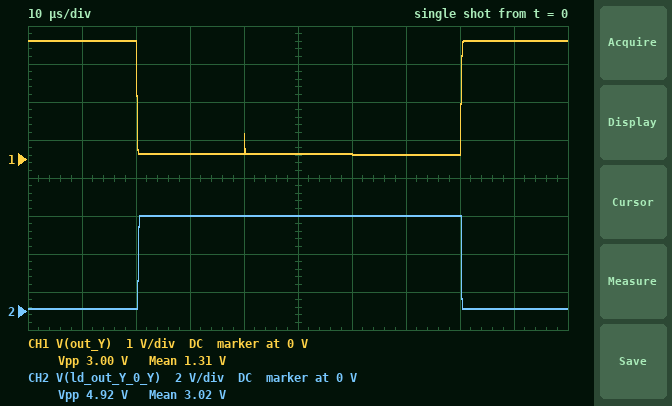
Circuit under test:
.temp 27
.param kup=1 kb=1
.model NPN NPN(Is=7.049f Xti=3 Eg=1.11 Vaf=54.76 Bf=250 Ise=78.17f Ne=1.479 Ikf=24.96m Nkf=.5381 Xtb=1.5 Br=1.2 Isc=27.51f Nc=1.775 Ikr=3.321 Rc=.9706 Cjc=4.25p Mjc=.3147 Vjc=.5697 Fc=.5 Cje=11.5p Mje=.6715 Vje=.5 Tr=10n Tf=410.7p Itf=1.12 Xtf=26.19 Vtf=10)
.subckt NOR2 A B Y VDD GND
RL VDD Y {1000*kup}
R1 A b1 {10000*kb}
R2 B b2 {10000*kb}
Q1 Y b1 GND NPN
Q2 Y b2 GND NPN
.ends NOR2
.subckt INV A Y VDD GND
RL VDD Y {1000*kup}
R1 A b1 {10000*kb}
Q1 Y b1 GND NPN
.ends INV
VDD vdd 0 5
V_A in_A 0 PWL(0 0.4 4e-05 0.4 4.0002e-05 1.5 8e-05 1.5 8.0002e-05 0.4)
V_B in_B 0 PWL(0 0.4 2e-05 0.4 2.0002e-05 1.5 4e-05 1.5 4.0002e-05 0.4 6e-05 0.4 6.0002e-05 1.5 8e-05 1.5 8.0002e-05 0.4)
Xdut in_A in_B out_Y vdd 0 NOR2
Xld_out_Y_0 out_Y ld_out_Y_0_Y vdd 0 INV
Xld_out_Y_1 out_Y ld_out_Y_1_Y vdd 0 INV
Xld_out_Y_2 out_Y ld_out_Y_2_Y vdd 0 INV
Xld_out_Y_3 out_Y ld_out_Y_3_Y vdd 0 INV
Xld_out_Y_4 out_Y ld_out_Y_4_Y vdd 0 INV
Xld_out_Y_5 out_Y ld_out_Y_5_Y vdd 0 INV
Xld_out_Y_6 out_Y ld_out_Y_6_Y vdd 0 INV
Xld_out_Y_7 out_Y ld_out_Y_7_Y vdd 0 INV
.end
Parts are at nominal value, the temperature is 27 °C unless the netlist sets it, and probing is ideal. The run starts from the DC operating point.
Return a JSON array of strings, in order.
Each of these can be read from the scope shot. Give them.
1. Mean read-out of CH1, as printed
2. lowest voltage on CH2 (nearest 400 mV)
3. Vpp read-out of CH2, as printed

["1.31 V", "0 V", "4.92 V"]
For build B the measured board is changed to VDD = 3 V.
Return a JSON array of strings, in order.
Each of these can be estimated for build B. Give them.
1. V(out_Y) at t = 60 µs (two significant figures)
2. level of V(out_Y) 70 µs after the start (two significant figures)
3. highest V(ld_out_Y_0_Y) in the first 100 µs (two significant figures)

["100 mV", "79 mV", "3.0 V"]
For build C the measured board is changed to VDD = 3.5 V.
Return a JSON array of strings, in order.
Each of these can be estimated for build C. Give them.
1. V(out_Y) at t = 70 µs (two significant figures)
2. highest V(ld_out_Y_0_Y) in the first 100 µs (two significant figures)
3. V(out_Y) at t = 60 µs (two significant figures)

["84 mV", "3.5 V", "110 mV"]
